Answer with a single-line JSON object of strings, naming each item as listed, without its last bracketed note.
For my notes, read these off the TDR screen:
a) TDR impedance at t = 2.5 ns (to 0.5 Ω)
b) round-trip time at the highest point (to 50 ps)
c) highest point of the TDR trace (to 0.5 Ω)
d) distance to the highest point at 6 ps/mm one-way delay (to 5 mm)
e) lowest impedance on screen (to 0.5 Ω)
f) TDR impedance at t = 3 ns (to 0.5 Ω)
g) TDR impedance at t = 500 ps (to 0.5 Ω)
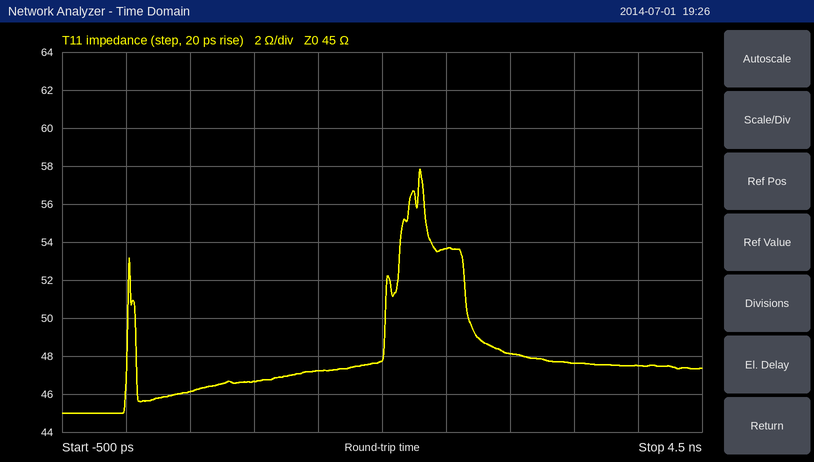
{"TDR impedance at t = 2.5 ns": "53.5 Ω", "round-trip time at the highest point": "2.30 ns", "highest point of the TDR trace": "58.0 Ω", "distance to the highest point at 6 ps/mm one-way delay": "190 mm", "lowest impedance on screen": "45.0 Ω", "TDR impedance at t = 3 ns": "48.0 Ω", "TDR impedance at t = 500 ps": "46.0 Ω"}
